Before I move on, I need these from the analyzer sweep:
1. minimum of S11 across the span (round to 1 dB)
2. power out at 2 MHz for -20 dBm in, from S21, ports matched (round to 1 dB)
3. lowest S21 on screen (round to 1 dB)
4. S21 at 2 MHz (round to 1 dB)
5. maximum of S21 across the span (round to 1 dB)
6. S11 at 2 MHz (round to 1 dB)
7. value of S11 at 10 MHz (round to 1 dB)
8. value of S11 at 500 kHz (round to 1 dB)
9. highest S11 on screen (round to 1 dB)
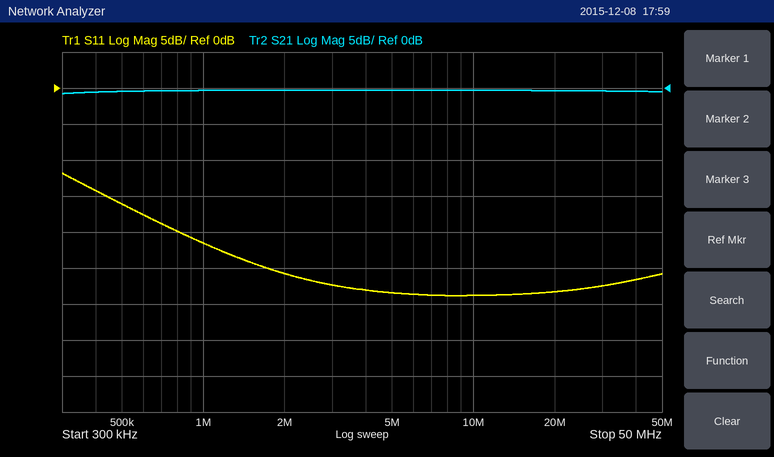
-29 dB
-20 dBm
-1 dB
0 dB
0 dB
-26 dB
-29 dB
-16 dB
-12 dB
